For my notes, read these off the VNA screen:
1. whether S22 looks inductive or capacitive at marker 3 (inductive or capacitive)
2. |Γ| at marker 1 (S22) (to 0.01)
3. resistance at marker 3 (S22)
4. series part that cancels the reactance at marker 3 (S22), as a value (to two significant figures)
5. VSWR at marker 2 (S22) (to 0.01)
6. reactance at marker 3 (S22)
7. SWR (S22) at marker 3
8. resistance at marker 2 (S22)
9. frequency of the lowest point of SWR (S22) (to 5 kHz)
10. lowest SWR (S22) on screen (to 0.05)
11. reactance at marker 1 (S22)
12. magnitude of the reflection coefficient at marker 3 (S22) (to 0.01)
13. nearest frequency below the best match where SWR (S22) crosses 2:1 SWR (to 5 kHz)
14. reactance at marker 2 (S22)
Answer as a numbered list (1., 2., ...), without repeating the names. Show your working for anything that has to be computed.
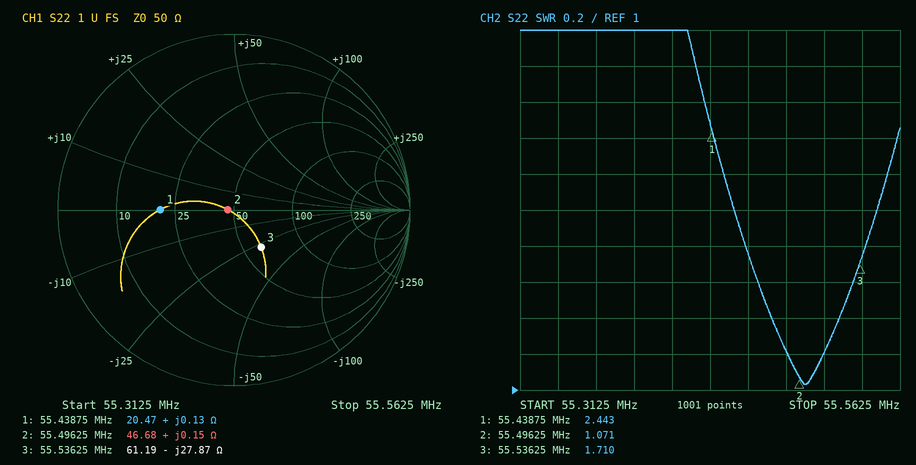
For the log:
1. capacitive
2. 0.42
3. 61.19 Ω
4. L = 27.87 Ω/(2π × 55.53625 MHz) ≈ 80 nH
5. 1.07
6. -27.87 Ω
7. 1.710
8. 46.68 Ω
9. 55.500 MHz
10. 1.05
11. +0.13 Ω
12. 0.26
13. 55.455 MHz
14. +0.15 Ω
